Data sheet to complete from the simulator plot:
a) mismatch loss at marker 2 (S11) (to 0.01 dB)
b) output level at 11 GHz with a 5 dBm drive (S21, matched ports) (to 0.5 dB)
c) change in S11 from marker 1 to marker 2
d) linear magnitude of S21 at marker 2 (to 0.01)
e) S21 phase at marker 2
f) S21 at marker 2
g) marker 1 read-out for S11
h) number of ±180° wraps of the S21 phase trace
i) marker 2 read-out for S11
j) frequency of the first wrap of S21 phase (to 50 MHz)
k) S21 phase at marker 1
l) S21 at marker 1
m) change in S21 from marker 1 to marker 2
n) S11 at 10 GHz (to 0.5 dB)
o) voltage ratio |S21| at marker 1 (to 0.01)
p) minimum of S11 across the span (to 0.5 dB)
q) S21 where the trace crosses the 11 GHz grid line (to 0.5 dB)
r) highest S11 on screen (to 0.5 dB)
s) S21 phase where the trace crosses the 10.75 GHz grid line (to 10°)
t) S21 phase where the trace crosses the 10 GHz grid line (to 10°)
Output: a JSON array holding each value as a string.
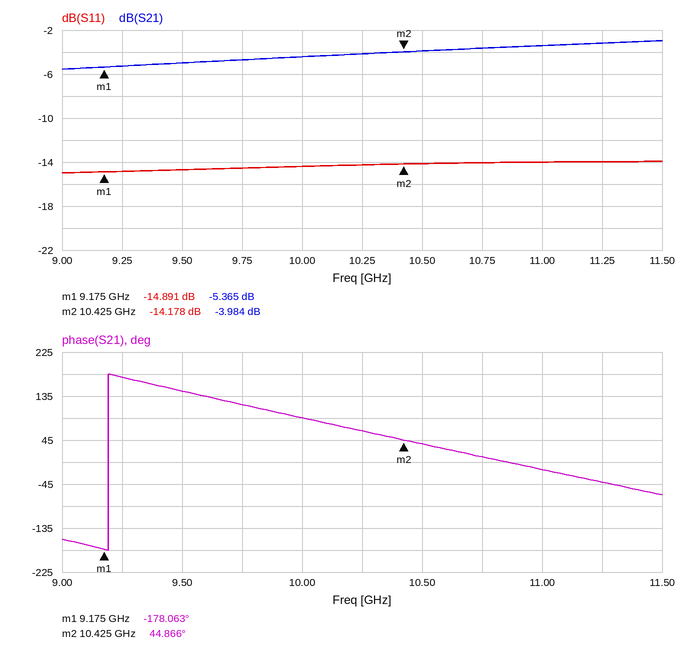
["0.17 dB", "1.5 dBm", "0.713 dB", "0.63", "44.866°", "-3.984 dB", "-14.891 dB", "1", "-14.178 dB", "9.20 GHz", "-178.063°", "-5.365 dB", "1.381 dB", "-14.5 dB", "0.54", "-15.0 dB", "-3.5 dB", "-14.0 dB", "10°", "90°"]
